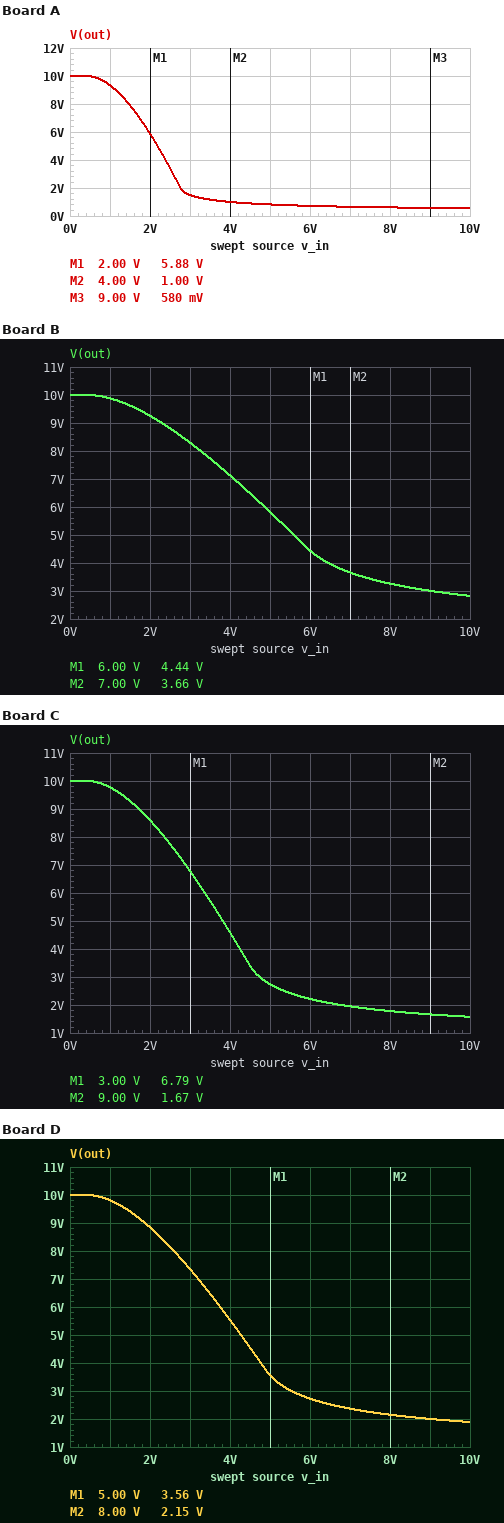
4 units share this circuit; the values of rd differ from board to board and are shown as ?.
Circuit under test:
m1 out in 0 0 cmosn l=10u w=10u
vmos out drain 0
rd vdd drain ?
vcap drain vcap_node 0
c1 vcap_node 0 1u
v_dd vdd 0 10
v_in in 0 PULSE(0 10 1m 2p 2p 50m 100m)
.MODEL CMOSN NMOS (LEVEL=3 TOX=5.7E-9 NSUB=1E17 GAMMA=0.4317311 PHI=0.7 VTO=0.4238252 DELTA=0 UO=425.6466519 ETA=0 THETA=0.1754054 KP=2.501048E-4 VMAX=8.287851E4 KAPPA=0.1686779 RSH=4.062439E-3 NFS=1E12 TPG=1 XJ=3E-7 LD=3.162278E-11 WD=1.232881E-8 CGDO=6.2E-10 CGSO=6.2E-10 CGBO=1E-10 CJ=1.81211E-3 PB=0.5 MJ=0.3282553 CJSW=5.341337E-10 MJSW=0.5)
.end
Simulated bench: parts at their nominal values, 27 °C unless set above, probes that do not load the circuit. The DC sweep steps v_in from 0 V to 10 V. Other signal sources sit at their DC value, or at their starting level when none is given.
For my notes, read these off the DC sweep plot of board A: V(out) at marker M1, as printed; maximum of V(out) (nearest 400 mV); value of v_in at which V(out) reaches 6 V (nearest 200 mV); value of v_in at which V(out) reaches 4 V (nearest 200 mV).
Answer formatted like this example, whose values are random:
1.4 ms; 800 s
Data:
5.88 V; 10.0 V; 2.0 V; 2.4 V
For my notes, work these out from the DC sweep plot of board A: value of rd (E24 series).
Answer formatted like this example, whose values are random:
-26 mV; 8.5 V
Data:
20 kΩ
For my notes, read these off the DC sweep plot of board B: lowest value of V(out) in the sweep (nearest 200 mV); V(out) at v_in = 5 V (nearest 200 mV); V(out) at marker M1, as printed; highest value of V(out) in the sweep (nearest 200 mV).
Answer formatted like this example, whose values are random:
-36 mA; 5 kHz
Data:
2.8 V; 5.8 V; 4.44 V; 10.0 V
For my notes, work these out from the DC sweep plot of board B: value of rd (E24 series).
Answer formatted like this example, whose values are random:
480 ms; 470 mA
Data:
3.6 kΩ
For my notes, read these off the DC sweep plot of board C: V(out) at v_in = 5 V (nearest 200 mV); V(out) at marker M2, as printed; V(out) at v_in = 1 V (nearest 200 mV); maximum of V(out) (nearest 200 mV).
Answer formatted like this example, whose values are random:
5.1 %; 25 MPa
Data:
2.8 V; 1.67 V; 9.8 V; 10.0 V
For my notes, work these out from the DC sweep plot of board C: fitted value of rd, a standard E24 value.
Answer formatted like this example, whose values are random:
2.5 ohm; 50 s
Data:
6.8 kΩ
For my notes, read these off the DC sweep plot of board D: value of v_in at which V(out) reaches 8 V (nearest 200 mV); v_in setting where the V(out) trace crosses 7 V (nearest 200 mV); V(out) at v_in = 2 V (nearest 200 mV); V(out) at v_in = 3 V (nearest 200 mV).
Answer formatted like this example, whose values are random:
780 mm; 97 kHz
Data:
2.6 V; 3.2 V; 8.8 V; 7.4 V
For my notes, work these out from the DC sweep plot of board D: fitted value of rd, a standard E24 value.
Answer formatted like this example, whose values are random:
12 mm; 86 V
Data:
5.6 kΩ
